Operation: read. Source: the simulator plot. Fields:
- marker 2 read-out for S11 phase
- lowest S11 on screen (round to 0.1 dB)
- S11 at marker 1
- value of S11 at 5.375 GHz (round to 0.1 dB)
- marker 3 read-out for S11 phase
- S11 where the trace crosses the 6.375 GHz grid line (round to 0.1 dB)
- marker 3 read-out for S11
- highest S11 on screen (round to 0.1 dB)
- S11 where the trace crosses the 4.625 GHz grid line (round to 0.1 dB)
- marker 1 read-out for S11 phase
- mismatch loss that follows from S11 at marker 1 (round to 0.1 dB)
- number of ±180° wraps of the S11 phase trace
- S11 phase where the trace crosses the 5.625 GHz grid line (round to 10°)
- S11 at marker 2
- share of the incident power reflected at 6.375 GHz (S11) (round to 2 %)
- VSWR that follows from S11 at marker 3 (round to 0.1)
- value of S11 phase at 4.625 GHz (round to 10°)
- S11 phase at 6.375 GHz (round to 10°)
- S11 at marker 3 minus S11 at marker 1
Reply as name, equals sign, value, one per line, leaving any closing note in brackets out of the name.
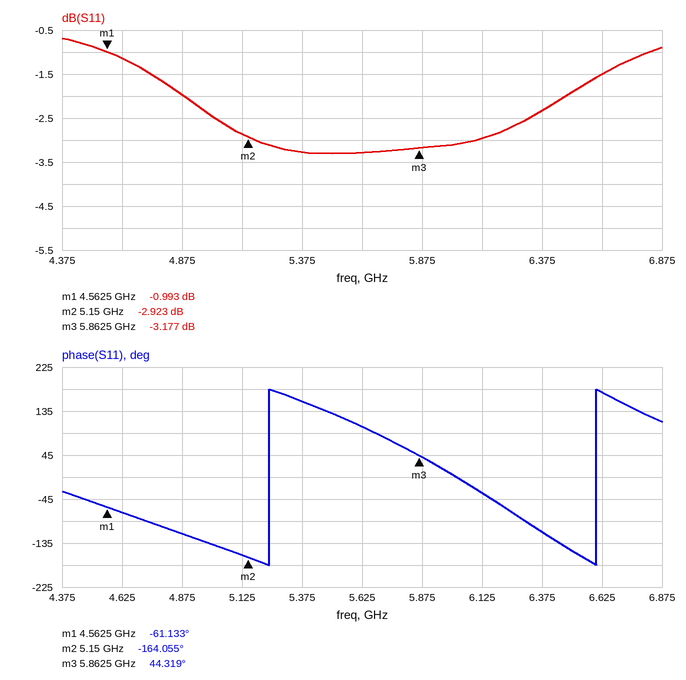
marker 2 read-out for S11 phase = -164.055°
lowest S11 on screen = -3.3 dB
S11 at marker 1 = -0.993 dB
value of S11 at 5.375 GHz = -3.3 dB
marker 3 read-out for S11 phase = 44.319°
S11 where the trace crosses the 6.375 GHz grid line = -2.3 dB
marker 3 read-out for S11 = -3.177 dB
highest S11 on screen = -0.7 dB
S11 where the trace crosses the 4.625 GHz grid line = -1.1 dB
marker 1 read-out for S11 phase = -61.133°
mismatch loss that follows from S11 at marker 1 = 6.9 dB
number of ±180° wraps of the S11 phase trace = 2
S11 phase where the trace crosses the 5.625 GHz grid line = 100°
S11 at marker 2 = -2.923 dB
share of the incident power reflected at 6.375 GHz (S11) = 58 %
VSWR that follows from S11 at marker 3 = 5.5
value of S11 phase at 4.625 GHz = -70°
S11 phase at 6.375 GHz = -110°
S11 at marker 3 minus S11 at marker 1 = -2.184 dB
